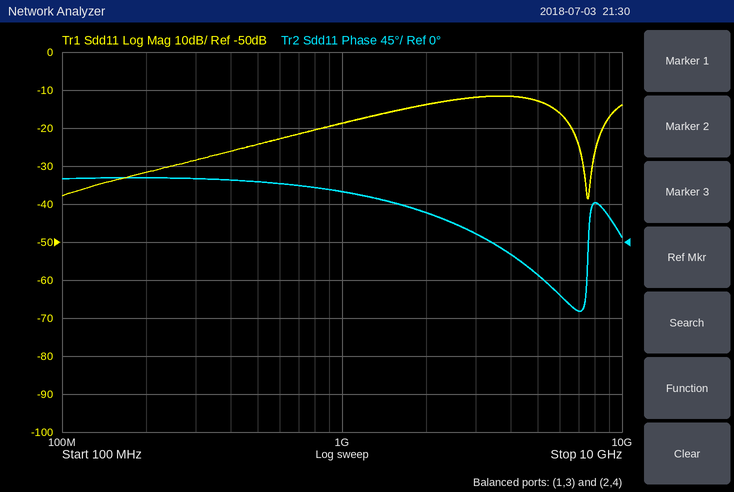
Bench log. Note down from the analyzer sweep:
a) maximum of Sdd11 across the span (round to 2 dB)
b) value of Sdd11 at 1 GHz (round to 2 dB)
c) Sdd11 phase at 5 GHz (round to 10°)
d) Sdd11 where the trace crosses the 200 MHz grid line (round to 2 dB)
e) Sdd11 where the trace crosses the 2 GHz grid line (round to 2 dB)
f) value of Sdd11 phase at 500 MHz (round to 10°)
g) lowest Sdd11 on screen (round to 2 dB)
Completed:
-12 dB
-18 dB
-40°
-32 dB
-14 dB
70°
-38 dB
